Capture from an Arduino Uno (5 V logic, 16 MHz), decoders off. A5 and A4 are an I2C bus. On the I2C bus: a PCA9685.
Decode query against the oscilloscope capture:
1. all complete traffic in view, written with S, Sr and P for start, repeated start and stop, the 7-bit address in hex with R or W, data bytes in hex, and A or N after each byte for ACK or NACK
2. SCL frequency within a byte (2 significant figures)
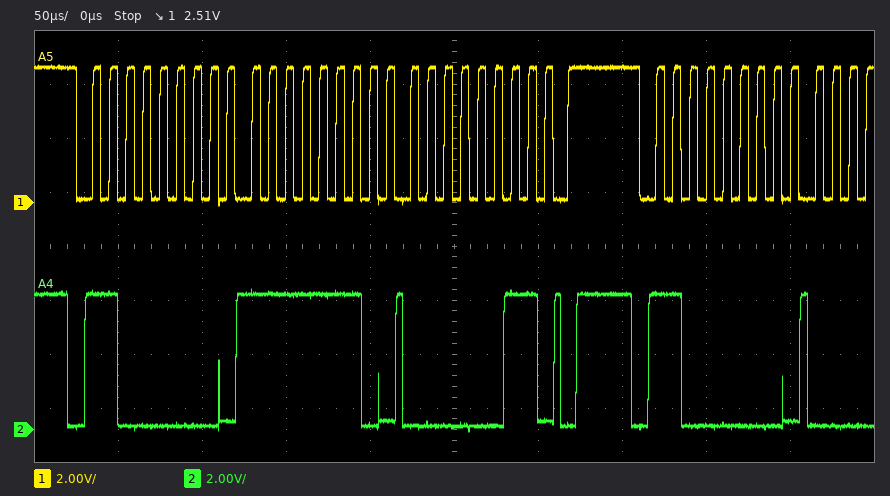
S 60W A FE A 03 A P S 60W A
100 kHz
